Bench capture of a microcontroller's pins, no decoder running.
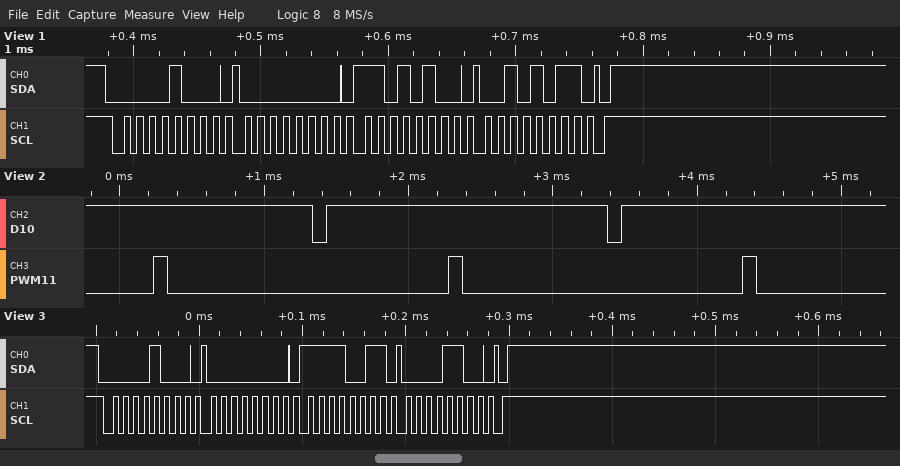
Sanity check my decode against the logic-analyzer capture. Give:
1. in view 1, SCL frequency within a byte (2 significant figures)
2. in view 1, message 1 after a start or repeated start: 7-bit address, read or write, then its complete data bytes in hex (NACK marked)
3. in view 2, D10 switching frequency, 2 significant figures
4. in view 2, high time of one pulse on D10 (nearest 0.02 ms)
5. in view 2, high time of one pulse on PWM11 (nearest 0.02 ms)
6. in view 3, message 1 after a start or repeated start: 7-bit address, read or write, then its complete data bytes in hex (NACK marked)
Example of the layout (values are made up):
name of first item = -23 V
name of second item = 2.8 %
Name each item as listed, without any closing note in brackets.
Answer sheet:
in view 1, SCL frequency within a byte = 100 kHz
in view 1, message 1 after a start or repeated start: 7-bit address, read or write, then its complete data bytes in hex = 0x04 write: 00 D4 2B
in view 2, D10 switching frequency, 2 significant figures = 490 Hz
in view 2, high time of one pulse on D10 = 1.94 ms
in view 2, high time of one pulse on PWM11 = 0.10 ms
in view 3, message 1 after a start or repeated start: 7-bit address, read or write, then its complete data bytes in hex = 0x04 write: 00 F3 0C
